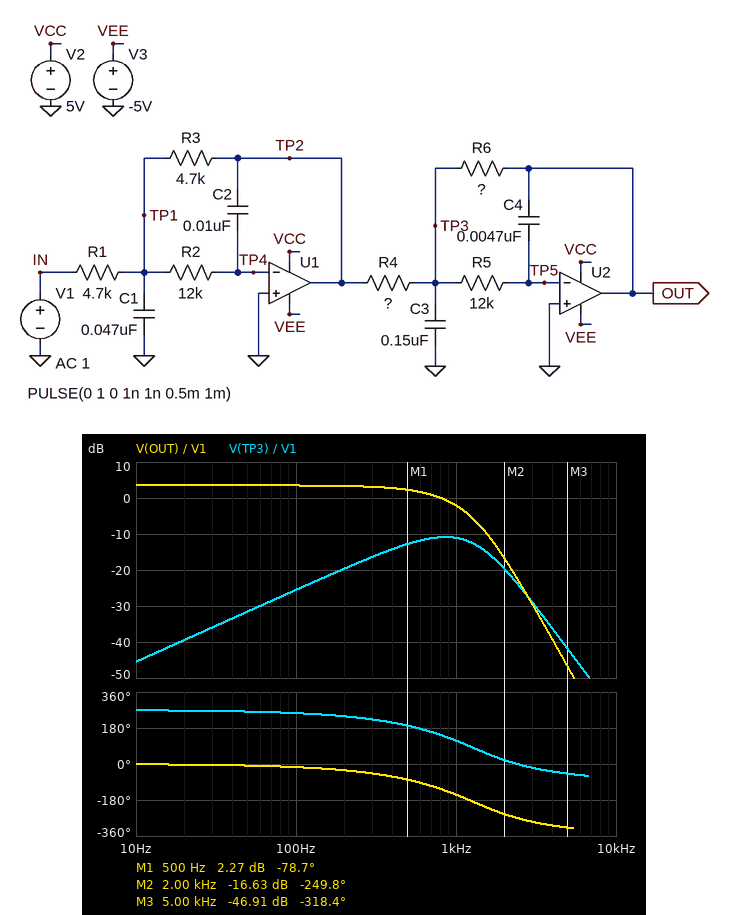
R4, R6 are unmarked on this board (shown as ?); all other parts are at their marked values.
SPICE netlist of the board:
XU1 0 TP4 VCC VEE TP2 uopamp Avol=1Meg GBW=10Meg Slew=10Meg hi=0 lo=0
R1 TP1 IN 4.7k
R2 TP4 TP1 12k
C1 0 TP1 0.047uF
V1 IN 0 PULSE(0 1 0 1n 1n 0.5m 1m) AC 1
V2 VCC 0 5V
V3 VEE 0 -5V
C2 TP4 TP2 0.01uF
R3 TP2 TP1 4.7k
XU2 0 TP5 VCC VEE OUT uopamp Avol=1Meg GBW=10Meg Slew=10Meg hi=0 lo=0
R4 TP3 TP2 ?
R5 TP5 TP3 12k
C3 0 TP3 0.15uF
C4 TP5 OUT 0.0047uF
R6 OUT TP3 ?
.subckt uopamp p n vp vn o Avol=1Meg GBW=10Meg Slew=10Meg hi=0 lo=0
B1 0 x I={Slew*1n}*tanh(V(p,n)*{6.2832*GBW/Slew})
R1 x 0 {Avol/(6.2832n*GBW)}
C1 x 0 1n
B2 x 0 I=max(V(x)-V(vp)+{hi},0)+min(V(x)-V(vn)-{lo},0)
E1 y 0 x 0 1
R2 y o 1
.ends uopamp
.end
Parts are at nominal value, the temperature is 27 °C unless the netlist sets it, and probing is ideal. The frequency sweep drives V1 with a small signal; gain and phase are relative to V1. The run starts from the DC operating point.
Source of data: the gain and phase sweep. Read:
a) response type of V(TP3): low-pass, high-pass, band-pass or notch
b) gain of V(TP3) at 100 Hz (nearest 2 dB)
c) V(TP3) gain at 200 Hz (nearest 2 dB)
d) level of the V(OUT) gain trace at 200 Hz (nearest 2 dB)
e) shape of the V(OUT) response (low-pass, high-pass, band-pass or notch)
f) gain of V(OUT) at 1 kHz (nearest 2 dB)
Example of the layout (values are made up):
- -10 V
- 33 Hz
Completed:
- band-pass
- -26 dB
- -20 dB
- 4 dB
- low-pass
- -2 dB
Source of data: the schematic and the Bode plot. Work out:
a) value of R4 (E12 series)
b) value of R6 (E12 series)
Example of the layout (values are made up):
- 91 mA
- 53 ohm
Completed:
- 1 kΩ
- 1.5 kΩ
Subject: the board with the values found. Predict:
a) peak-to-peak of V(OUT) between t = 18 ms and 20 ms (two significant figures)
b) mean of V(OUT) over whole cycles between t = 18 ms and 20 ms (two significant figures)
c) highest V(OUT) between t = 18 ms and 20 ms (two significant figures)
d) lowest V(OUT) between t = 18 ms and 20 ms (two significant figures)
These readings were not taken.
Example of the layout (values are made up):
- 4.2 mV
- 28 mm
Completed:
- 1.0 V
- 750 mV
- 1.3 V
- 240 mV
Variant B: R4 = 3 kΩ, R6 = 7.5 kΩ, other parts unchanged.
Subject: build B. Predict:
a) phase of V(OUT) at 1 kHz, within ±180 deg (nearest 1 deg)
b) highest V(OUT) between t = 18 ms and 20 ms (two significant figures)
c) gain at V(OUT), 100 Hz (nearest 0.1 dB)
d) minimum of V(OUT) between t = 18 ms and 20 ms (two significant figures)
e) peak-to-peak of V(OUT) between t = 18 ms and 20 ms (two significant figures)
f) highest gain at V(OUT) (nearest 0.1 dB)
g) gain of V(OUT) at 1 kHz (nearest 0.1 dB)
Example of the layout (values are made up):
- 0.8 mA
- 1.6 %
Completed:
- 133 deg
- 1.7 V
- 8.0 dB
- 830 mV
- 840 mV
- 8.7 dB
- -3.6 dB
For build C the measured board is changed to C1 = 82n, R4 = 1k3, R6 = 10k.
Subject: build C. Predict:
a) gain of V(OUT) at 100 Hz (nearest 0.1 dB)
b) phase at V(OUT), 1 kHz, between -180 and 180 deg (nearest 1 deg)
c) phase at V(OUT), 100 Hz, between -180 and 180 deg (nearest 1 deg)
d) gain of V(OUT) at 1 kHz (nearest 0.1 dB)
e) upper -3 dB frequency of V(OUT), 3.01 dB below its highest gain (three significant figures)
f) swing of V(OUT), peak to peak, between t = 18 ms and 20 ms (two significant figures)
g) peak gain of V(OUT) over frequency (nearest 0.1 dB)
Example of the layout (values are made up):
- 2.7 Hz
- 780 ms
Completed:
- 17.5 dB
- 121 deg
- -30 deg
- -0.5 dB
- 389 Hz
- 1.2 V
- 17.7 dB
